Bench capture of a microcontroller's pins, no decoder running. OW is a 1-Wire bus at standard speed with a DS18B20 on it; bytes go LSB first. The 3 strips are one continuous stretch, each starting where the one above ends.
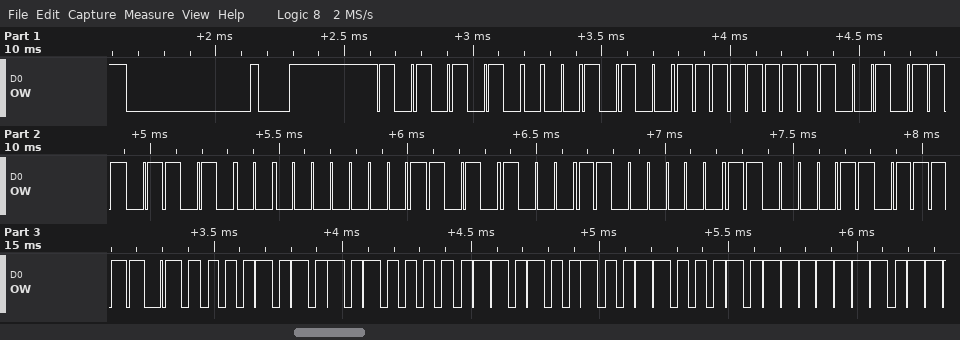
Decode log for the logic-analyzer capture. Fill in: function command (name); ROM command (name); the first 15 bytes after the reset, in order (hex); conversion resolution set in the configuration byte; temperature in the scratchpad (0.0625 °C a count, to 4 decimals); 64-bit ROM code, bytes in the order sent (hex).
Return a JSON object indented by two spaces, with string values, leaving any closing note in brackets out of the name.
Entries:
{
  "function command": "Read Scratchpad",
  "ROM command": "Match ROM",
  "the first 15 bytes after the reset, in order": "55 28 FF E9 16 80 15 03 C3 BE 50 05 4B 46 7F",
  "conversion resolution set in the configuration byte": "12 bits",
  "temperature in the scratchpad": "85.0000 °C",
  "64-bit ROM code, bytes in the order sent": "28 FF E9 16 80 15 03 C3"
}
